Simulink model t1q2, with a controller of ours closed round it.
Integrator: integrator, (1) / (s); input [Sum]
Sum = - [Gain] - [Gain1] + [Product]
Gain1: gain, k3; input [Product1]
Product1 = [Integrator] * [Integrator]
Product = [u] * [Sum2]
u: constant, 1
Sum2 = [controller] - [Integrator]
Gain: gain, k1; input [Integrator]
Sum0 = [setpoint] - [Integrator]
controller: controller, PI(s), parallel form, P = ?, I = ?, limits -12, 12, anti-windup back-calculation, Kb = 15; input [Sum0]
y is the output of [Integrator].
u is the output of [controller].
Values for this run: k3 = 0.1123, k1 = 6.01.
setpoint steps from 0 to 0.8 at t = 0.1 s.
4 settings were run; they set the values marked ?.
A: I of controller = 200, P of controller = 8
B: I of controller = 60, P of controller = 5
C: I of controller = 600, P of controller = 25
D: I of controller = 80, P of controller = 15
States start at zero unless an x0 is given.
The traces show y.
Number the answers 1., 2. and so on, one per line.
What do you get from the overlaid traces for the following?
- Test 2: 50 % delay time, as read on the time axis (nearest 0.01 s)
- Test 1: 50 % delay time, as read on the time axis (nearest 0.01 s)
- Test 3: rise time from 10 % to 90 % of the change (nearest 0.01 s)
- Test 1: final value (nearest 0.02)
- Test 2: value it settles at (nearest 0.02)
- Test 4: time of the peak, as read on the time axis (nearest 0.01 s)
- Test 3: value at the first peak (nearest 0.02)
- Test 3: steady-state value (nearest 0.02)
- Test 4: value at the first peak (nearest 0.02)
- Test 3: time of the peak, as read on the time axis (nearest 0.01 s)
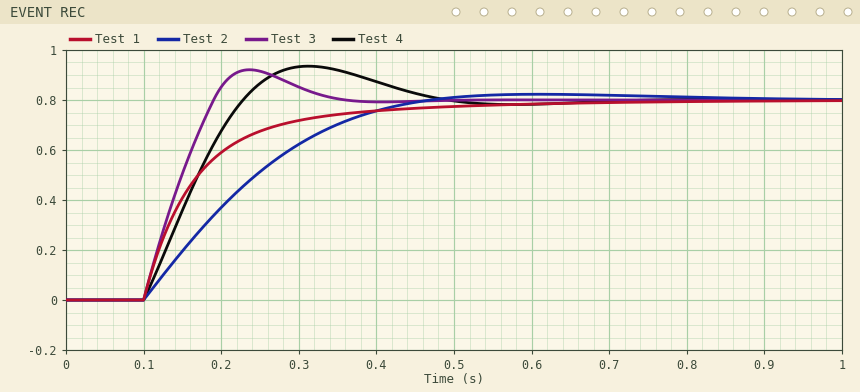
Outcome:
1. 0.21 s
2. 0.15 s
3. 0.07 s
4. 0.80
5. 0.80
6. 0.31 s
7. 0.92
8. 0.80
9. 0.94
10. 0.24 s
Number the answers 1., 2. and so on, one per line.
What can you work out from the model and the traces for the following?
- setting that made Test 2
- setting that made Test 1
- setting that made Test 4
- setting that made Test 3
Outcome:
1. B
2. D
3. A
4. C
